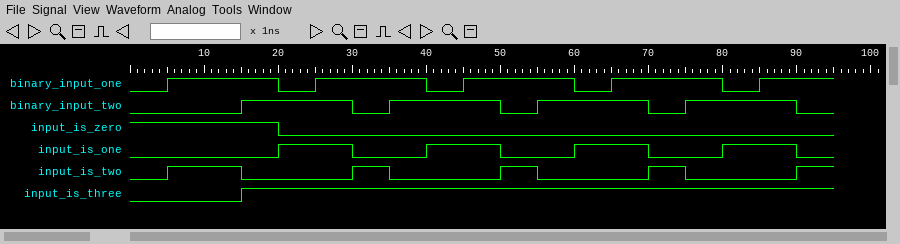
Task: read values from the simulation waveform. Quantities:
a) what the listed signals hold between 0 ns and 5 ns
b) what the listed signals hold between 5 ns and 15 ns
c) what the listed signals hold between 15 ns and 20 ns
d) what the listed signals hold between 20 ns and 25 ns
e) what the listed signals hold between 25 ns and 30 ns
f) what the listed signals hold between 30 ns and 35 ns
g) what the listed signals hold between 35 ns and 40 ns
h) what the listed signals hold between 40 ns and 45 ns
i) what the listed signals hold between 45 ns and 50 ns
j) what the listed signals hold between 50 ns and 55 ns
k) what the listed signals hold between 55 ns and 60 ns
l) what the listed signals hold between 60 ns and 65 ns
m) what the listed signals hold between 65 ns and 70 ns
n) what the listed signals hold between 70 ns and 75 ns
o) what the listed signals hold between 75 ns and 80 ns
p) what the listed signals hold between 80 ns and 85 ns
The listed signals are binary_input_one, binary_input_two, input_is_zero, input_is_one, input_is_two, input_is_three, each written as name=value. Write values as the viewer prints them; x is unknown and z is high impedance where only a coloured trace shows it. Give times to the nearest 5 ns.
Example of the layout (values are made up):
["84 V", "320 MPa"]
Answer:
["binary_input_one=0, binary_input_two=0, input_is_zero=1, input_is_one=0, input_is_two=0, input_is_three=0", "binary_input_one=1, binary_input_two=0, input_is_zero=1, input_is_one=0, input_is_two=1, input_is_three=0", "binary_input_one=1, binary_input_two=1, input_is_zero=1, input_is_one=0, input_is_two=0, input_is_three=1", "binary_input_one=0, binary_input_two=1, input_is_zero=0, input_is_one=1, input_is_two=0, input_is_three=1", "binary_input_one=1, binary_input_two=1, input_is_zero=0, input_is_one=1, input_is_two=0, input_is_three=1", "binary_input_one=1, binary_input_two=0, input_is_zero=0, input_is_one=0, input_is_two=1, input_is_three=1", "binary_input_one=1, binary_input_two=1, input_is_zero=0, input_is_one=0, input_is_two=0, input_is_three=1", "binary_input_one=0, binary_input_two=1, input_is_zero=0, input_is_one=1, input_is_two=0, input_is_three=1", "binary_input_one=1, binary_input_two=1, input_is_zero=0, input_is_one=1, input_is_two=0, input_is_three=1", "binary_input_one=1, binary_input_two=0, input_is_zero=0, input_is_one=0, input_is_two=1, input_is_three=1", "binary_input_one=1, binary_input_two=1, input_is_zero=0, input_is_one=0, input_is_two=0, input_is_three=1", "binary_input_one=0, binary_input_two=1, input_is_zero=0, input_is_one=1, input_is_two=0, input_is_three=1", "binary_input_one=1, binary_input_two=1, input_is_zero=0, input_is_one=1, input_is_two=0, input_is_three=1", "binary_input_one=1, binary_input_two=0, input_is_zero=0, input_is_one=0, input_is_two=1, input_is_three=1", "binary_input_one=1, binary_input_two=1, input_is_zero=0, input_is_one=0, input_is_two=0, input_is_three=1", "binary_input_one=0, binary_input_two=1, input_is_zero=0, input_is_one=1, input_is_two=0, input_is_three=1"]
